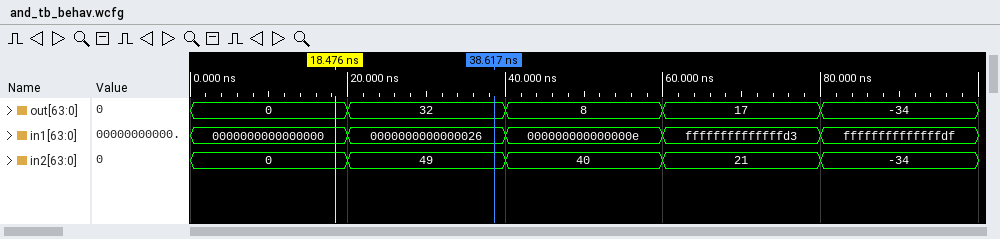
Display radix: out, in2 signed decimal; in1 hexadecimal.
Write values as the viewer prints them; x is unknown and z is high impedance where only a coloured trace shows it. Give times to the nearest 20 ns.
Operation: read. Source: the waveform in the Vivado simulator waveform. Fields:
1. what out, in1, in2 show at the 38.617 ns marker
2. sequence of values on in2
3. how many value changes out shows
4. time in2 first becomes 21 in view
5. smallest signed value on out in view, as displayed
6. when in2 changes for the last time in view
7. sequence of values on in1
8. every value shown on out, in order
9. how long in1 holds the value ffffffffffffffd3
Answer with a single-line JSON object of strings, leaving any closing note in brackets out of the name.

{"what out, in1, in2 show at the 38.617 ns marker": "out=32, in1=0000000000000026, in2=49", "sequence of values on in2": "0, 49, 40, 21, -34", "how many value changes out shows": "4", "time in2 first becomes 21 in view": "60 ns", "smallest signed value on out in view, as displayed": "-34", "when in2 changes for the last time in view": "80 ns", "sequence of values on in1": "0000000000000000, 0000000000000026, 000000000000000e, ffffffffffffffd3, ffffffffffffffdf", "every value shown on out, in order": "0, 32, 8, 17, -34", "how long in1 holds the value ffffffffffffffd3": "20 ns"}
